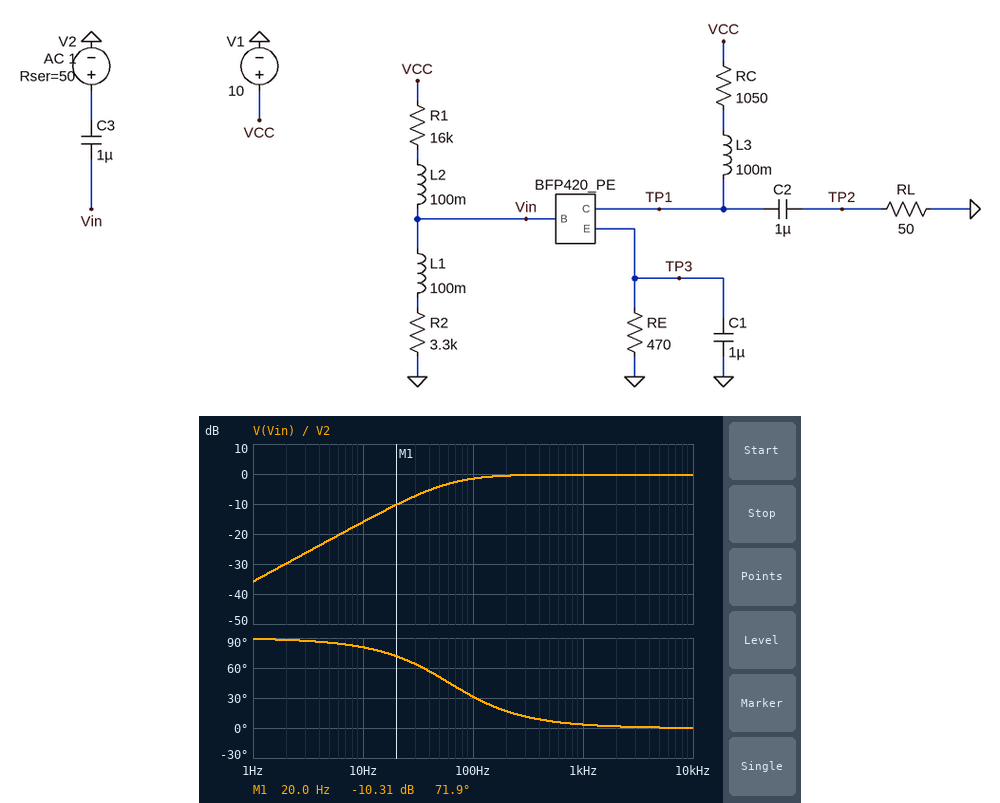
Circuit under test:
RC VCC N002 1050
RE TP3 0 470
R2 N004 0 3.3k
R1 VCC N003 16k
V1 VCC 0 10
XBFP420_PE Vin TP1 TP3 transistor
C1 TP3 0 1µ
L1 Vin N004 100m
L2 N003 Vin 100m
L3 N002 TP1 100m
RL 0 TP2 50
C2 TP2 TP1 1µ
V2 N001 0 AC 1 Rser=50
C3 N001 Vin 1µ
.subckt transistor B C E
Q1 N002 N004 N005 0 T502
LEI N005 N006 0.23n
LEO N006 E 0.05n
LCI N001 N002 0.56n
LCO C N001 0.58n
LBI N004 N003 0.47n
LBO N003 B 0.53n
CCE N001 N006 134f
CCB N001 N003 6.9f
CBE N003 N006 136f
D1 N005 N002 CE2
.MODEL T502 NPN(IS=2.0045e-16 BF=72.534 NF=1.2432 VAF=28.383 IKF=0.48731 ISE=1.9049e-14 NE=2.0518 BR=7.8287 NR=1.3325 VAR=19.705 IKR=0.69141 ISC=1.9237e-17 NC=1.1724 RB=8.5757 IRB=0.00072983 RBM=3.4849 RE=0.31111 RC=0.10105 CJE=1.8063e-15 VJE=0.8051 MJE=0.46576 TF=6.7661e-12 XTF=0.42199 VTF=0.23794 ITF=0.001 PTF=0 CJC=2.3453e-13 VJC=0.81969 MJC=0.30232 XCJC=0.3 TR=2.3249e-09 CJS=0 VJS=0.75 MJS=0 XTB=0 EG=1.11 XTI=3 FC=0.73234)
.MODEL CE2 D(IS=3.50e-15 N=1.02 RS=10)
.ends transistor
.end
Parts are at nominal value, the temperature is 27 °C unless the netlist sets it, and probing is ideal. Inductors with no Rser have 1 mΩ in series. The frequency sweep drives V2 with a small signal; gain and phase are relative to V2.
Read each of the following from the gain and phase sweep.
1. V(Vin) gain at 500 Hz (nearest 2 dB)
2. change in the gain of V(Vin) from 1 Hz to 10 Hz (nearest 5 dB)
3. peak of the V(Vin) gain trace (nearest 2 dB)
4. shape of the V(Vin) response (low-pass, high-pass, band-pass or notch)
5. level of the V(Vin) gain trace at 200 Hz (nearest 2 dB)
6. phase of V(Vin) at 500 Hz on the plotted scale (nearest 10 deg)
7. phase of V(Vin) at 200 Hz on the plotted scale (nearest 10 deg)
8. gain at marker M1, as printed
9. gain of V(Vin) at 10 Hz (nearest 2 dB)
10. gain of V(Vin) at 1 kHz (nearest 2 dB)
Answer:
0 dB
20 dB
0 dB
high-pass
0 dB
10 deg
20 deg
-10.31 dB
-16 dB
0 dB
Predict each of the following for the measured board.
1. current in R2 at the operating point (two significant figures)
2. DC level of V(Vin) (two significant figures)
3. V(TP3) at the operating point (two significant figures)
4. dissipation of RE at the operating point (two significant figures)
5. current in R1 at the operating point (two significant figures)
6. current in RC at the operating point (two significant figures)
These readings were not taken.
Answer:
500 µA
1.7 V
710 mV
1.1 mW
520 µA
1.5 mA
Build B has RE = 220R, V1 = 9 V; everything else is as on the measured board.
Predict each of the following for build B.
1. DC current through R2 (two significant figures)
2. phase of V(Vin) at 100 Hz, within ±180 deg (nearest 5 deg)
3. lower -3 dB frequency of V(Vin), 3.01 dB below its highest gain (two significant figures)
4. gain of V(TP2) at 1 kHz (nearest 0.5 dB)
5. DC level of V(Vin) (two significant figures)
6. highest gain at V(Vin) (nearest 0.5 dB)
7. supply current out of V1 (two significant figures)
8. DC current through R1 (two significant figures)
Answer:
440 µA
35 deg
66 Hz
-9.0 dB
1.5 V
0 dB
2.7 mA
470 µA
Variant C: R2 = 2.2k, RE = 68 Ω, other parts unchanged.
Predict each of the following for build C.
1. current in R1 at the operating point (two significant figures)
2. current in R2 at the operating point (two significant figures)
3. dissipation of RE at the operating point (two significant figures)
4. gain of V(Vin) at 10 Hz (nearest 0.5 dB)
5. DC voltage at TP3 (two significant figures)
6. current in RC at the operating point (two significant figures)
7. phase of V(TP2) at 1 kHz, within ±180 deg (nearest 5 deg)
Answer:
550 µA
520 µA
470 µW
-20.5 dB
180 mV
2.6 mA
-145 deg
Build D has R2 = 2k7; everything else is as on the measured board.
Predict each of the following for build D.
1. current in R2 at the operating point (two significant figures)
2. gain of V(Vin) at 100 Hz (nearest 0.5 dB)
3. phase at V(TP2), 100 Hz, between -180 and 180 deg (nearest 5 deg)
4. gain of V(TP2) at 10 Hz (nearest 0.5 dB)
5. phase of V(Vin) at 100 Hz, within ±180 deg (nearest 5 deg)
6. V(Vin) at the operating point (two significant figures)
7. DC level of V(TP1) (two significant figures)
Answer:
520 µA
-2.0 dB
-70 deg
-61.0 dB
35 deg
1.4 V
8.9 V
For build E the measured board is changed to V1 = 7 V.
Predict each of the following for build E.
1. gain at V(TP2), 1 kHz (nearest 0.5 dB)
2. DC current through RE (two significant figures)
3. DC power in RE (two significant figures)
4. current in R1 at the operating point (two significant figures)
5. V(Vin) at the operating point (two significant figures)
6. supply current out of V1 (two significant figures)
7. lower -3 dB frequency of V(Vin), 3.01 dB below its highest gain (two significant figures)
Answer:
-11.0 dB
550 µA
140 µW
360 µA
1.2 V
910 µA
62 Hz
